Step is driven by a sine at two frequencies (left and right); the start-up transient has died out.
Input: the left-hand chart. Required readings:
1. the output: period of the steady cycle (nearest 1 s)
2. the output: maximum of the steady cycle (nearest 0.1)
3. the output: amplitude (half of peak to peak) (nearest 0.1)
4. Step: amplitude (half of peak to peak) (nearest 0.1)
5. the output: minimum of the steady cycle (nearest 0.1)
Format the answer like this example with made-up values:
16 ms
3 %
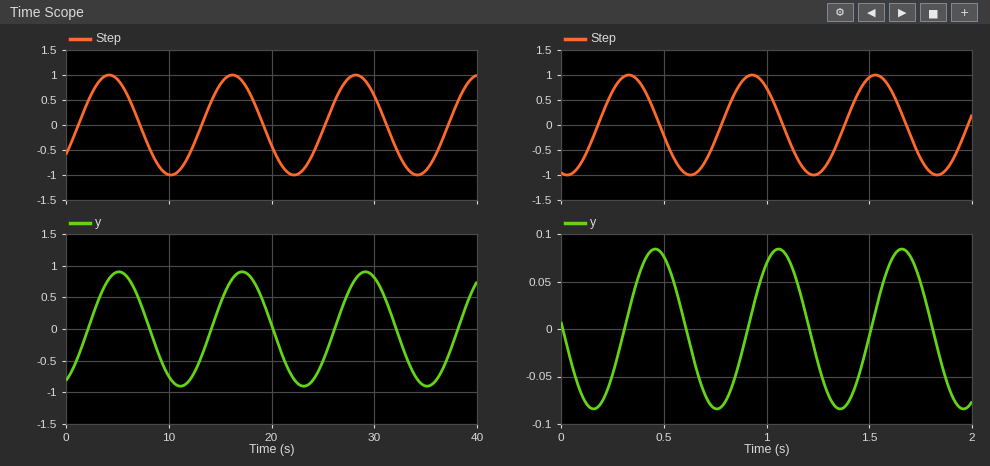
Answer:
12 s
0.9
0.9
1.0
-0.9
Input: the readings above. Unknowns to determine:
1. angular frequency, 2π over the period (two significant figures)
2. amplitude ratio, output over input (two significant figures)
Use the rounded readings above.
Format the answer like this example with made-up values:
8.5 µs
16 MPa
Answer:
0.52 rad/s
0.90
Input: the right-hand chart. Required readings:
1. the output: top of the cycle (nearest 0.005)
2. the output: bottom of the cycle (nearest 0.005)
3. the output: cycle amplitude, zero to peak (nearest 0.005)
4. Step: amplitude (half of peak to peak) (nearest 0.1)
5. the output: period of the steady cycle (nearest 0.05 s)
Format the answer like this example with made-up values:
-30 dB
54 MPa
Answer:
0.085
-0.085
0.085
1.0
0.60 s
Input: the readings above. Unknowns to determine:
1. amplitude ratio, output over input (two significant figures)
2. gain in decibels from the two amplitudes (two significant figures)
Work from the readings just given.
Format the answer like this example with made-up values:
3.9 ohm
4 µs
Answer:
0.085
-21 dB
